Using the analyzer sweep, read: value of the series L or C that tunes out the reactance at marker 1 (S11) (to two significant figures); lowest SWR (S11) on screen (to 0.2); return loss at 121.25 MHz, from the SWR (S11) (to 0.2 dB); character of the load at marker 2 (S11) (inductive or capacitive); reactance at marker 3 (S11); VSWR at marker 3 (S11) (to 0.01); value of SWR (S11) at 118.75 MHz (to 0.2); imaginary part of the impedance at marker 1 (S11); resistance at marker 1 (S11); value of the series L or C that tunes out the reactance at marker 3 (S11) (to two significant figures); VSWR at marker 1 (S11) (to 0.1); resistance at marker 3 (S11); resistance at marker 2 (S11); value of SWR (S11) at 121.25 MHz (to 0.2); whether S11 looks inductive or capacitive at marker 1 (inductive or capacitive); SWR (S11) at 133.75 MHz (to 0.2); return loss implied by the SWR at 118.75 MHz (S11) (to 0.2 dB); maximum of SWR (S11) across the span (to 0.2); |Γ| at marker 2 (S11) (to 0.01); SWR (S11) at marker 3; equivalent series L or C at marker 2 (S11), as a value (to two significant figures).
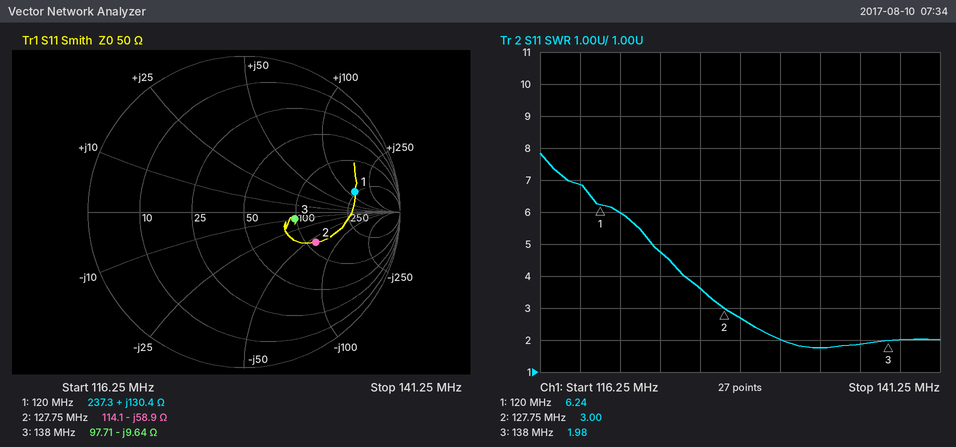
10 pF
1.8
3.0 dB
capacitive
-9.64 Ω
1.98
6.8
+130.4 Ω
237.3 Ω
11 nH
6.2
97.71 Ω
114.1 Ω
6.0
inductive
1.8
2.6 dB
7.8
0.50
1.98
21 pF
